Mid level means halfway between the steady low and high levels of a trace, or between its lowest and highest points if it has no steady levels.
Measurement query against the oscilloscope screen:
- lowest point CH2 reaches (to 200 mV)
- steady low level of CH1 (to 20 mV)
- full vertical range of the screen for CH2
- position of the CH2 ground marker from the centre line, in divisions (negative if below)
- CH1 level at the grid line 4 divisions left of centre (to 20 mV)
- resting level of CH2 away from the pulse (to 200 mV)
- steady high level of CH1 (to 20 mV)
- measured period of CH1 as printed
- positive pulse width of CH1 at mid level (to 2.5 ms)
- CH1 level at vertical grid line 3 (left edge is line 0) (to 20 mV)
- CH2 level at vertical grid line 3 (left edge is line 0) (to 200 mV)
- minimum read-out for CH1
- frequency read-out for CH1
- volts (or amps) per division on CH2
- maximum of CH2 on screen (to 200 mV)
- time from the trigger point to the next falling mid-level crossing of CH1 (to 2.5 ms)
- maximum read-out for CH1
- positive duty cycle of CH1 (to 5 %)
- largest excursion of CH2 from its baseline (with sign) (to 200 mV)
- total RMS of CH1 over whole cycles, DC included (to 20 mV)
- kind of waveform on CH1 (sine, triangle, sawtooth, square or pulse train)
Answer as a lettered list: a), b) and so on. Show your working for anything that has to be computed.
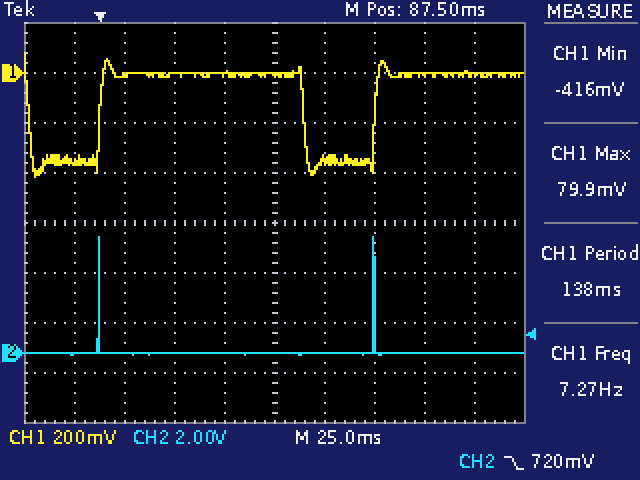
a) 0.0 V
b) -360 mV
c) 16 V
d) -2.6 div
e) -360 mV
f) 0.0 V
g) 0 mV
h) 138 ms
i) 102.5 ms
j) 0 mV
k) 0.0 V
l) -416 mV
m) 7.27 Hz
n) 2 V
o) 4.6 V
p) 102.5 ms
q) 79.9 mV
r) 75 %
s) 4.6 V − (0.0 V) = +4.6 V
t) √(0.75 × (0 mV)² + 0.25 × (-360 mV)²) ≈ 180 mV
u) pulse train
